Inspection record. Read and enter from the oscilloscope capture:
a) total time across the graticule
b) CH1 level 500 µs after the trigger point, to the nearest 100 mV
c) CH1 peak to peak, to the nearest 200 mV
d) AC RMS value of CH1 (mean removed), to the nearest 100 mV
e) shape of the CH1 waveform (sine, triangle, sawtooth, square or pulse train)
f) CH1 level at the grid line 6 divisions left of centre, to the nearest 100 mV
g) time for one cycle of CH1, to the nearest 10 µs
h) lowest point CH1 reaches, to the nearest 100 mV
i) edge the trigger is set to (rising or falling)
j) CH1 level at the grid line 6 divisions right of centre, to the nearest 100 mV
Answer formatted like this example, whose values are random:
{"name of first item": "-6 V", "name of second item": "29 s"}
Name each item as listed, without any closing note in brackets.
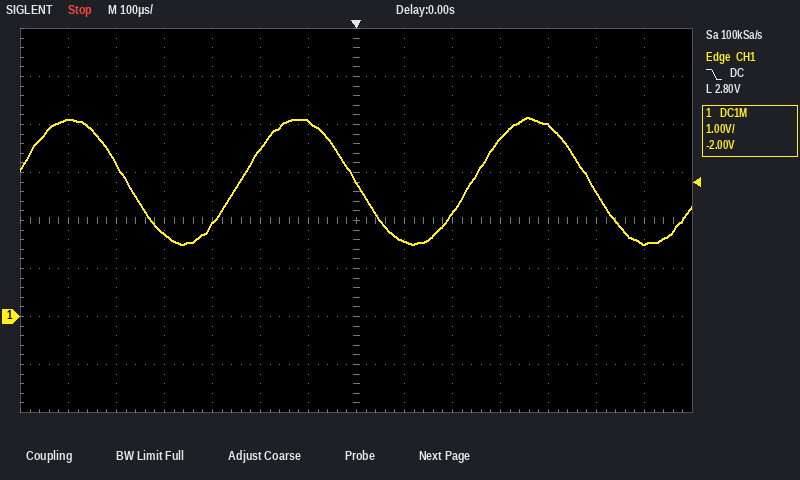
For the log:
{"total time across the graticule": "1.4 ms", "CH1 level 500 µs after the trigger point, to the nearest 100 mV": "2.6 V", "CH1 peak to peak, to the nearest 200 mV": "2.6 V", "AC RMS value of CH1 (mean removed), to the nearest 100 mV": "900 mV", "shape of the CH1 waveform": "sine", "CH1 level at the grid line 6 divisions left of centre, to the nearest 100 mV": "4.1 V", "time for one cycle of CH1, to the nearest 10 µs": "480 µs", "lowest point CH1 reaches, to the nearest 100 mV": "1.5 V", "edge the trigger is set to": "falling", "CH1 level at the grid line 6 divisions right of centre, to the nearest 100 mV": "1.5 V"}
